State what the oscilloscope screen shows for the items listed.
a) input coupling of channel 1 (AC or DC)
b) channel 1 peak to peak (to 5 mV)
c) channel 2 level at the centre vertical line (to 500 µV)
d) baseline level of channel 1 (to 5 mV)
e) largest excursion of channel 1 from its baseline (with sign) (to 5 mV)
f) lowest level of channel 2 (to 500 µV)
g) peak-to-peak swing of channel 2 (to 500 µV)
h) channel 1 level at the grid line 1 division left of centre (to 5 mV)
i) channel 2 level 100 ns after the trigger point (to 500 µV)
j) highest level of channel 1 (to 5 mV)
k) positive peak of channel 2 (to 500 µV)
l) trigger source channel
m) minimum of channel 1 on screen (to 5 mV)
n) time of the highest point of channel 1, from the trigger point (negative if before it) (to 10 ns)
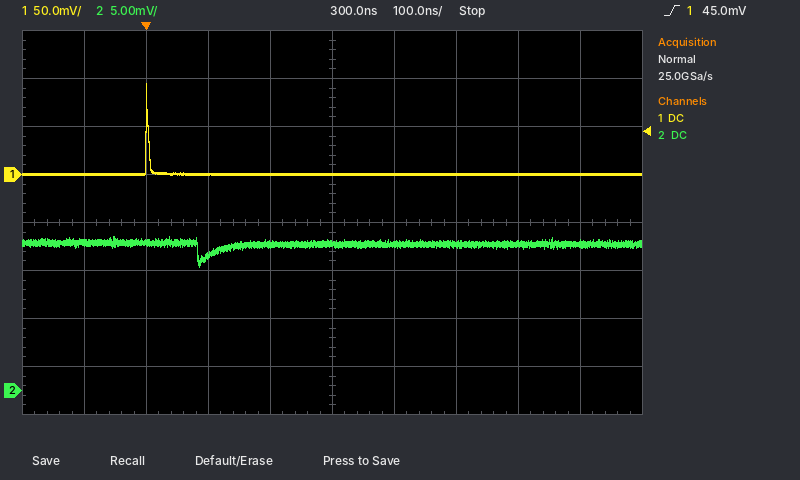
DC
95 mV
15.5 mV
0 mV
+95 mV
13.0 mV
3.0 mV
0 mV
14.0 mV
95 mV
16.0 mV
channel 1
0 mV
0 ns
